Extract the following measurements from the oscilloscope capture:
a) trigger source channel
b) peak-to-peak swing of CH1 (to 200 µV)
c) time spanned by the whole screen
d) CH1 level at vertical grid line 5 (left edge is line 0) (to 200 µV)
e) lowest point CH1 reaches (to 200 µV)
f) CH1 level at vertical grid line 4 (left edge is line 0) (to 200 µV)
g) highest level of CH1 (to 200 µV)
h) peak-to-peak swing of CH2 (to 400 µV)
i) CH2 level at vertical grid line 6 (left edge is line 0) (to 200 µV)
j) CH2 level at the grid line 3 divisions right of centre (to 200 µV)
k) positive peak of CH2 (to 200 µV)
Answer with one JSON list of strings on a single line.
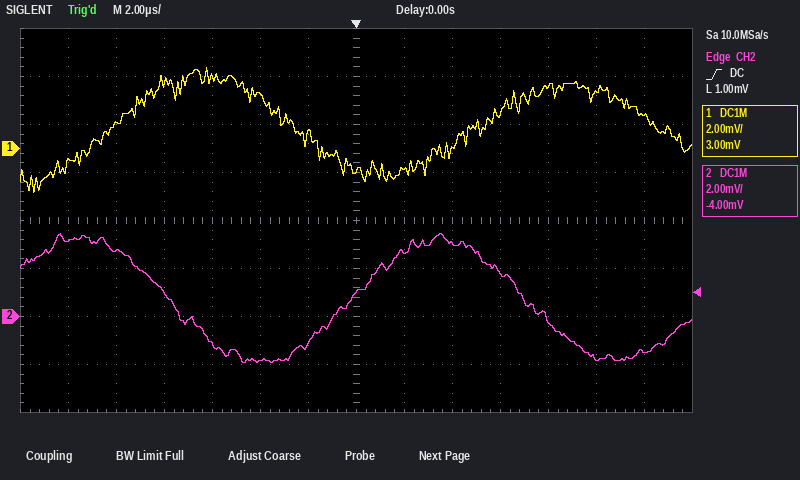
["CH2", "5.2 mV", "28 µs", "2.2 mV", "-1.8 mV", "3.0 mV", "3.4 mV", "5.2 mV", "-1.2 mV", "1.8 mV", "3.4 mV"]
